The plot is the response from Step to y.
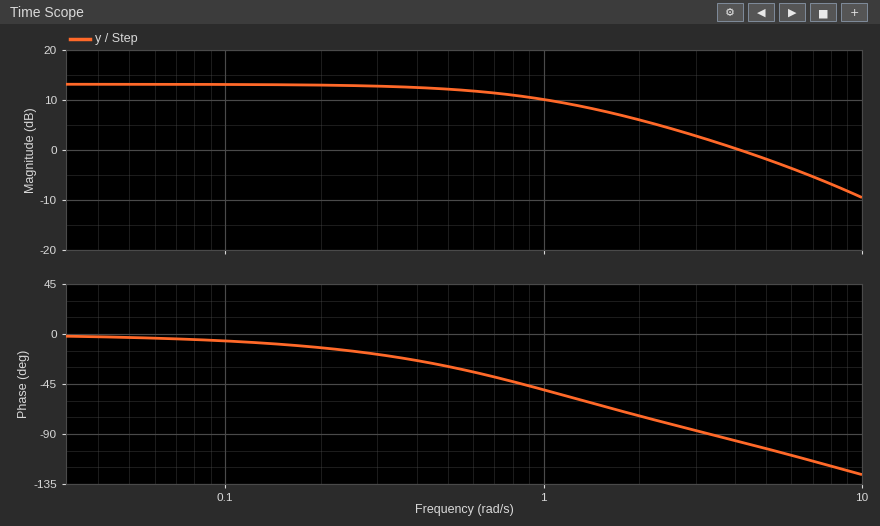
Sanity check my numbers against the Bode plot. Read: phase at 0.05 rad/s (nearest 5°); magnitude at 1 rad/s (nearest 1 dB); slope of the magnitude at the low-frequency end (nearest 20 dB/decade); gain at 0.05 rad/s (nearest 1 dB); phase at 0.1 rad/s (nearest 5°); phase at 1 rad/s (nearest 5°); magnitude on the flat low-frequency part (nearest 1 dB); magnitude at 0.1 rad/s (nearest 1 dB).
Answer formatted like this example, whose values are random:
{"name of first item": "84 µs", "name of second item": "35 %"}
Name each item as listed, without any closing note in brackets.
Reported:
{"phase at 0.05 rad/s": "-5°", "magnitude at 1 rad/s": "10 dB", "slope of the magnitude at the low-frequency end": "0 dB/decade", "gain at 0.05 rad/s": "13 dB", "phase at 0.1 rad/s": "-5°", "phase at 1 rad/s": "-50°", "magnitude on the flat low-frequency part": "13 dB", "magnitude at 0.1 rad/s": "13 dB"}
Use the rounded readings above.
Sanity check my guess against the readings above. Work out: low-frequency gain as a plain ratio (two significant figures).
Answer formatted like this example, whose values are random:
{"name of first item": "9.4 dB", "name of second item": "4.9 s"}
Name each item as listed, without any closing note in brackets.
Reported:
{"low-frequency gain as a plain ratio": "4.5"}
